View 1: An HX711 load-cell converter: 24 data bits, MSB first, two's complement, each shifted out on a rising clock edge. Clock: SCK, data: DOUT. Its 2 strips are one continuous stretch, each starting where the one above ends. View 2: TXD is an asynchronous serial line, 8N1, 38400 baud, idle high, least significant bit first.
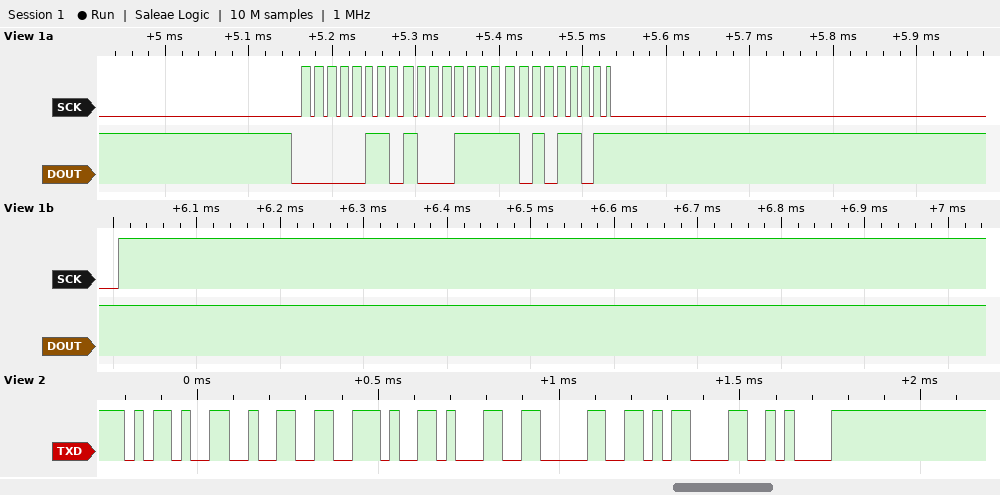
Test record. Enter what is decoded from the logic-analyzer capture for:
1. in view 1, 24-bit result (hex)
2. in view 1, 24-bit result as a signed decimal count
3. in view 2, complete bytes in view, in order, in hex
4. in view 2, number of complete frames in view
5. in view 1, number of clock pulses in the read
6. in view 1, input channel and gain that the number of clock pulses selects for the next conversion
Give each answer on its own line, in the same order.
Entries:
0x068FAD
429997
2D 32 2E 31 30 0D 0A
7
26
channel B, gain 32
